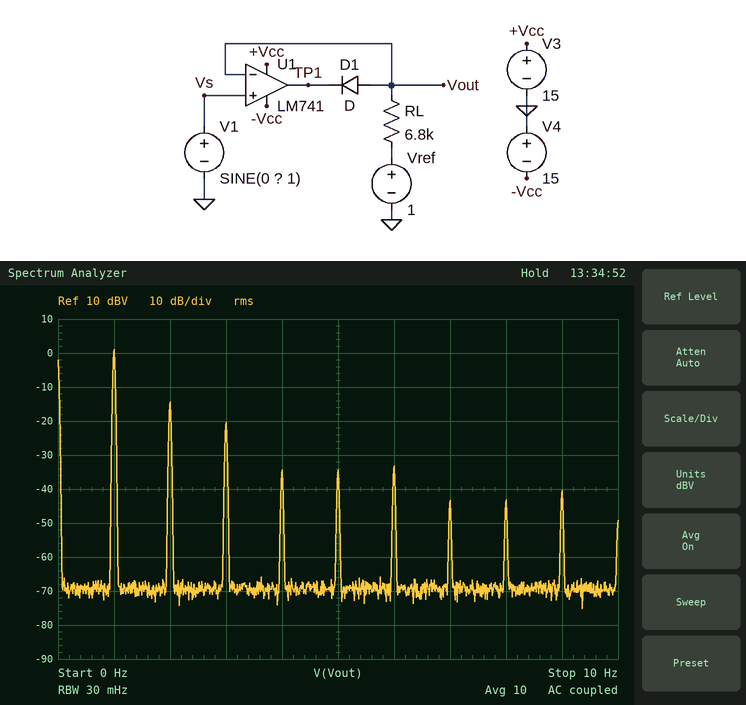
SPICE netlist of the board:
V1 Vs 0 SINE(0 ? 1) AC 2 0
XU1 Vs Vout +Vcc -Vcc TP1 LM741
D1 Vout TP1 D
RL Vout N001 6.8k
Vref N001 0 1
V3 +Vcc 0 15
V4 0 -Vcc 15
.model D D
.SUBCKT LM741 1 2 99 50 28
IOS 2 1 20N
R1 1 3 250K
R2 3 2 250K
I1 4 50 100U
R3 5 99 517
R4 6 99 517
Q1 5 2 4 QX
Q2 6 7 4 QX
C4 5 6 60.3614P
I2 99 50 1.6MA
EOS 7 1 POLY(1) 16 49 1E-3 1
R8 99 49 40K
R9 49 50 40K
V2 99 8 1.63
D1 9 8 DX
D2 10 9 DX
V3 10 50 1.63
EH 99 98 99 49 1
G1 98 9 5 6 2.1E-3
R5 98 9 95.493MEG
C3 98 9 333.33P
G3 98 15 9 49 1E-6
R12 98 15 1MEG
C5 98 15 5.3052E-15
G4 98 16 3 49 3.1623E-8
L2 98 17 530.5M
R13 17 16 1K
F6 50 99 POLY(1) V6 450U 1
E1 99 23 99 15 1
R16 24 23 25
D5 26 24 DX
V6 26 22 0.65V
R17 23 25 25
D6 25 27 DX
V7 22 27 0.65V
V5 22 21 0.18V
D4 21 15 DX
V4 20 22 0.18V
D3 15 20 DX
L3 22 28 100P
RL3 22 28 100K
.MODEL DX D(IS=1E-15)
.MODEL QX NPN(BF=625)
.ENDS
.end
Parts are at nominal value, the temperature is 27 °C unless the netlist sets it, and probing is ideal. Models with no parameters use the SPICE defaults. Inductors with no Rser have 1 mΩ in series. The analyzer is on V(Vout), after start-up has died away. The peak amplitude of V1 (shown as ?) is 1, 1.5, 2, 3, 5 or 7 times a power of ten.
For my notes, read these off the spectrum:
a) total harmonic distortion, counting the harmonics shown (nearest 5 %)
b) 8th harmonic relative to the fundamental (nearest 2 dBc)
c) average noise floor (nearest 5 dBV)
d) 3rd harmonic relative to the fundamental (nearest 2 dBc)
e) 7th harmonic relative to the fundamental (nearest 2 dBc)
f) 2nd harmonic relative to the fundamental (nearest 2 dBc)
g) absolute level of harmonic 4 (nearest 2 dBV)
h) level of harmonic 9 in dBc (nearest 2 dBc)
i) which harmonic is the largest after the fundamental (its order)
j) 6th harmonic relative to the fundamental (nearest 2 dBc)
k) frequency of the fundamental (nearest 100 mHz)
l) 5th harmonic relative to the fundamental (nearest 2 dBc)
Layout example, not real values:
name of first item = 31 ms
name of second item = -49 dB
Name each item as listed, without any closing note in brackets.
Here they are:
total harmonic distortion, counting the harmonics shown = 20 %
8th harmonic relative to the fundamental = -44 dBc
average noise floor = -70 dBV
3rd harmonic relative to the fundamental = -22 dBc
7th harmonic relative to the fundamental = -44 dBc
2nd harmonic relative to the fundamental = -16 dBc
absolute level of harmonic 4 = -34 dBV
level of harmonic 9 in dBc = -42 dBc
which harmonic is the largest after the fundamental = 2
6th harmonic relative to the fundamental = -34 dBc
frequency of the fundamental = 1.0 Hz
5th harmonic relative to the fundamental = -36 dBc
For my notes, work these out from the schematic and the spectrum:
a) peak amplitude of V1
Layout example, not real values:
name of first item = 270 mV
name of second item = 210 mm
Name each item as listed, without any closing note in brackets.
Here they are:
peak amplitude of V1 = 2 V
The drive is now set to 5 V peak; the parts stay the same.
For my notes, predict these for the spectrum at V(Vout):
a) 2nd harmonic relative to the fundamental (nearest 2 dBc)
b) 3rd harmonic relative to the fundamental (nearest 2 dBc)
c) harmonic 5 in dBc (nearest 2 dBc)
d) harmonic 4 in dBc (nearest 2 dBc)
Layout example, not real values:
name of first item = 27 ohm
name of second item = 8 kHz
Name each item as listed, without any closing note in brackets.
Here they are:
2nd harmonic relative to the fundamental = -10 dBc
3rd harmonic relative to the fundamental = -24 dBc
harmonic 5 in dBc = -30 dBc
harmonic 4 in dBc = -26 dBc
